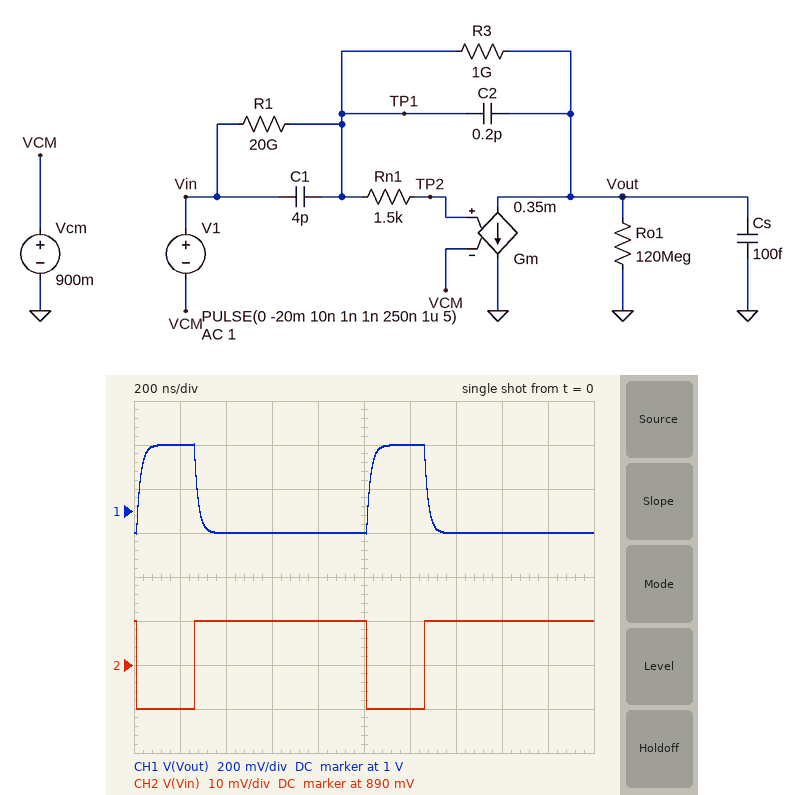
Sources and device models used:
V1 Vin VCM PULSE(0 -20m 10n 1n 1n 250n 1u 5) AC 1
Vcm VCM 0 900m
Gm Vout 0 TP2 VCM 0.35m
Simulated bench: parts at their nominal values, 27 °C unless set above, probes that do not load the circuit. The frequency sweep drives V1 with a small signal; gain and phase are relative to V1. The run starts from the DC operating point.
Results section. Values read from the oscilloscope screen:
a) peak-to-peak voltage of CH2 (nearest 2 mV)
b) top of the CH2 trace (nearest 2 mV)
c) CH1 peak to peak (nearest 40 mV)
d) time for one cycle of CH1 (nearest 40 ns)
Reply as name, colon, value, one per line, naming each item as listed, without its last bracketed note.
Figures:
peak-to-peak voltage of CH2: 20 mV
top of the CH2 trace: 900 mV
CH1 peak to peak: 400 mV
time for one cycle of CH1: 1.00 µs
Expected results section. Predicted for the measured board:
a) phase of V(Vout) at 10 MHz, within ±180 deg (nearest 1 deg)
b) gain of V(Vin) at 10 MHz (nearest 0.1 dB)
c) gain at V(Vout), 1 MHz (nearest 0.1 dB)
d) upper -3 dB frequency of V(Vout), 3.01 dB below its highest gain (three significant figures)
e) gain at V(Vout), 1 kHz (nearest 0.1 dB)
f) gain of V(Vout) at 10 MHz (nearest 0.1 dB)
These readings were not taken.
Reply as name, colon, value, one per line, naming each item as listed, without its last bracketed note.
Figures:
phase of V(Vout) at 10 MHz, within ±180 deg: 130 deg
gain of V(Vin) at 10 MHz: 0 dB
gain at V(Vout), 1 MHz: 26.0 dB
upper -3 dB frequency of V(Vout), 3.01 dB below its highest gain: 9.15 MHz
gain at V(Vout), 1 kHz: 23.9 dB
gain of V(Vout) at 10 MHz: 22.6 dB
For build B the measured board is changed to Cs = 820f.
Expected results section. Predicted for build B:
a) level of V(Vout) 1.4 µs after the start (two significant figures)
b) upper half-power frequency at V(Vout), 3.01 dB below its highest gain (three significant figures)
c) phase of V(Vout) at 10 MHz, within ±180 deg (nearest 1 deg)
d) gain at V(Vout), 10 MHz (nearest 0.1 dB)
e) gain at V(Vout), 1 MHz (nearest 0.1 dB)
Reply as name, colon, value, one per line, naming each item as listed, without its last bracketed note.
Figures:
level of V(Vout) 1.4 µs after the start: 940 mV
upper half-power frequency at V(Vout), 3.01 dB below its highest gain: 2.63 MHz
phase of V(Vout) at 10 MHz, within ±180 deg: 103 deg
gain at V(Vout), 10 MHz: 14.1 dB
gain at V(Vout), 1 MHz: 25.4 dB
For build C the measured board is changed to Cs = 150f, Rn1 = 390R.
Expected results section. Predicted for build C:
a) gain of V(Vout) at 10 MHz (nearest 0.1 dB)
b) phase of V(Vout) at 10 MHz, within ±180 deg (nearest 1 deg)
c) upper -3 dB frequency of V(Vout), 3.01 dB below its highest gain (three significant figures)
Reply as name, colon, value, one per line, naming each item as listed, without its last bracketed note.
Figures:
gain of V(Vout) at 10 MHz: 21.8 dB
phase of V(Vout) at 10 MHz, within ±180 deg: 126 deg
upper -3 dB frequency of V(Vout), 3.01 dB below its highest gain: 7.80 MHz
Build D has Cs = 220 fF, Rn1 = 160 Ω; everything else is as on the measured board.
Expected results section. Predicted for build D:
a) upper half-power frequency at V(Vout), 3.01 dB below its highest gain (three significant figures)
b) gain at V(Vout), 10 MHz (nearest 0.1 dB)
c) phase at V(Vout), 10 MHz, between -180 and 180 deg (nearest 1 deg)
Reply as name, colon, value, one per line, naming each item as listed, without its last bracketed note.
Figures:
upper half-power frequency at V(Vout), 3.01 dB below its highest gain: 6.47 MHz
gain at V(Vout), 10 MHz: 20.7 dB
phase at V(Vout), 10 MHz, between -180 and 180 deg: 121 deg
